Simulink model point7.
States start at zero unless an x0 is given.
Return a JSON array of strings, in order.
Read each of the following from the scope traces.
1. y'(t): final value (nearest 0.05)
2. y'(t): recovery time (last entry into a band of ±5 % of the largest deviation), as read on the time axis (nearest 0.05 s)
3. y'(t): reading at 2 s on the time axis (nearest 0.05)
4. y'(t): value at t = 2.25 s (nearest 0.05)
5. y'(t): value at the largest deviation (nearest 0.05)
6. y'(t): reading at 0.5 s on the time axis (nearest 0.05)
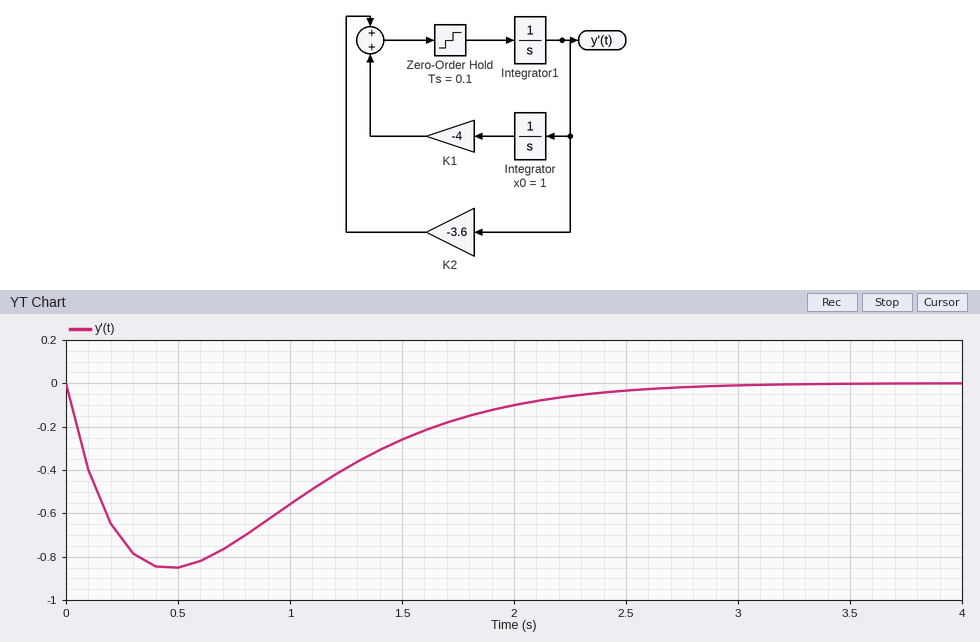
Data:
["0.00", "2.40 s", "-0.10", "-0.05", "-0.85", "-0.85"]
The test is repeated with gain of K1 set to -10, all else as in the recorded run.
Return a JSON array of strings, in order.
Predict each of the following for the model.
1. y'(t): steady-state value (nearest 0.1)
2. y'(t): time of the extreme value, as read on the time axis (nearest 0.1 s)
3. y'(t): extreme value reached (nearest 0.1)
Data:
["0.0", "0.3 s", "-1.8"]
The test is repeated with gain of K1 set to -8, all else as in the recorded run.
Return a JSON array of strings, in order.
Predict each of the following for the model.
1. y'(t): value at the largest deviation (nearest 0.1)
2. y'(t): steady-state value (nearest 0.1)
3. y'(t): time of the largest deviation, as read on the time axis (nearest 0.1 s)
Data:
["-1.5", "0.0", "0.4 s"]
